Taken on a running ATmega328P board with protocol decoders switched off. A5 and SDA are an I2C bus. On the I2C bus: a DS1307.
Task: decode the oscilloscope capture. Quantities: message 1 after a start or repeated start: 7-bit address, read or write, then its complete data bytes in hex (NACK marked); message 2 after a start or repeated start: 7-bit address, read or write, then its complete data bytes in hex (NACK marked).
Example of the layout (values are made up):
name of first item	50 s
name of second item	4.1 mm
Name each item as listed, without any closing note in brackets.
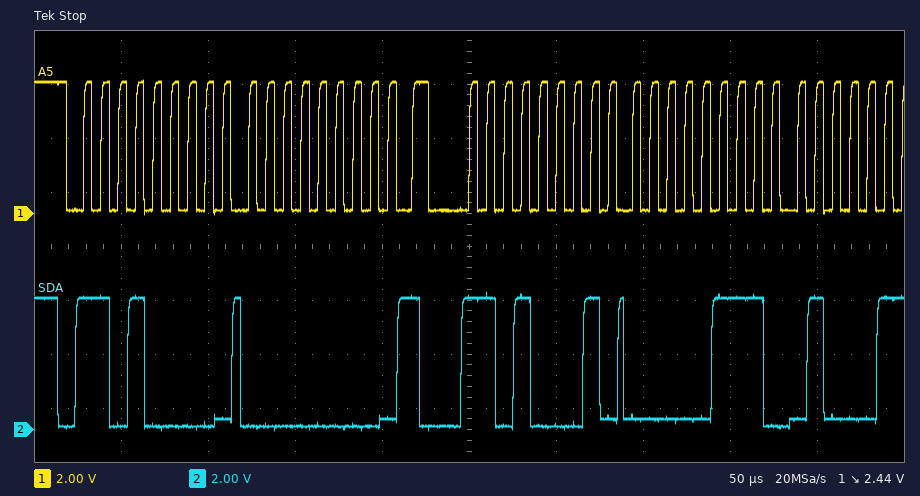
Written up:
message 1 after a start or repeated start: 7-bit address, read or write, then its complete data bytes in hex	0x68 write: 00
message 2 after a start or repeated start: 7-bit address, read or write, then its complete data bytes in hex	0x68 read: 07
